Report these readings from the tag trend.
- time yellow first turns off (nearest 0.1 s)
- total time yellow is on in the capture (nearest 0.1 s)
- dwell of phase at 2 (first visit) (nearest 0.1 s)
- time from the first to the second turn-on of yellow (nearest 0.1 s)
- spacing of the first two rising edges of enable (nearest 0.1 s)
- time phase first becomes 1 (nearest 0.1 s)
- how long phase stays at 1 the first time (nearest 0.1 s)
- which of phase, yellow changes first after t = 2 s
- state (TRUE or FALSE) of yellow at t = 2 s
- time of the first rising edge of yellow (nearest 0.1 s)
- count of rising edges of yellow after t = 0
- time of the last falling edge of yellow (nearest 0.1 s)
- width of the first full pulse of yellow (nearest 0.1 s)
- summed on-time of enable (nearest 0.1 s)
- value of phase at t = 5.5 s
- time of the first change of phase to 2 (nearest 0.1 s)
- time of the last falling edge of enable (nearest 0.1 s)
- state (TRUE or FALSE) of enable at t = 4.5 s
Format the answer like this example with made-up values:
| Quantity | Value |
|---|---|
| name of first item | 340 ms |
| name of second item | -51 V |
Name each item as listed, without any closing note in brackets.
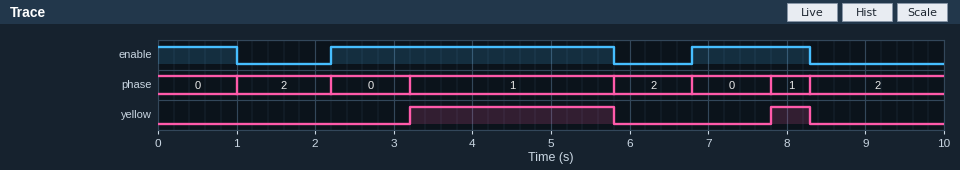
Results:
| Quantity | Value |
|---|---|
| time yellow first turns off | 5.8 s |
| total time yellow is on in the capture | 3.1 s |
| dwell of phase at 2 (first visit) | 1.2 s |
| time from the first to the second turn-on of yellow | 4.6 s |
| spacing of the first two rising edges of enable | 4.6 s |
| time phase first becomes 1 | 3.2 s |
| how long phase stays at 1 the first time | 2.6 s |
| which of phase, yellow changes first after t = 2 s | phase |
| state (TRUE or FALSE) of yellow at t = 2 s | FALSE |
| time of the first rising edge of yellow | 3.2 s |
| count of rising edges of yellow after t = 0 | 2 |
| time of the last falling edge of yellow | 8.3 s |
| width of the first full pulse of yellow | 2.6 s |
| summed on-time of enable | 6.1 s |
| value of phase at t = 5.5 s | 1 |
| time of the first change of phase to 2 | 1.0 s |
| time of the last falling edge of enable | 8.3 s |
| state (TRUE or FALSE) of enable at t = 4.5 s | TRUE |
